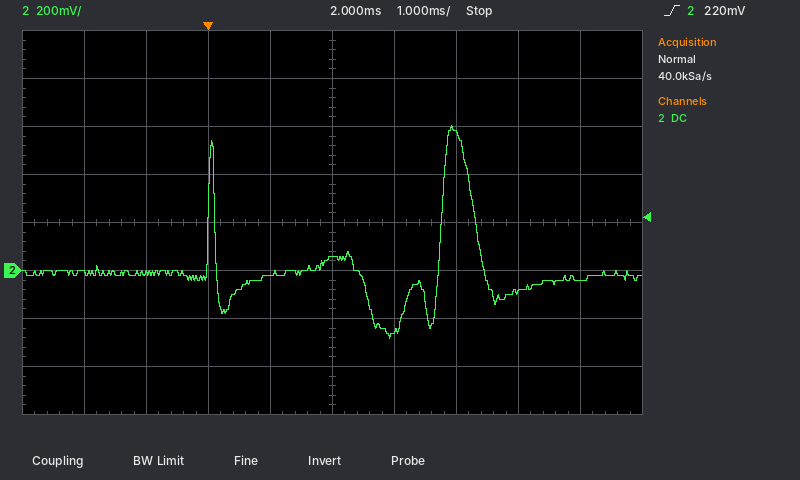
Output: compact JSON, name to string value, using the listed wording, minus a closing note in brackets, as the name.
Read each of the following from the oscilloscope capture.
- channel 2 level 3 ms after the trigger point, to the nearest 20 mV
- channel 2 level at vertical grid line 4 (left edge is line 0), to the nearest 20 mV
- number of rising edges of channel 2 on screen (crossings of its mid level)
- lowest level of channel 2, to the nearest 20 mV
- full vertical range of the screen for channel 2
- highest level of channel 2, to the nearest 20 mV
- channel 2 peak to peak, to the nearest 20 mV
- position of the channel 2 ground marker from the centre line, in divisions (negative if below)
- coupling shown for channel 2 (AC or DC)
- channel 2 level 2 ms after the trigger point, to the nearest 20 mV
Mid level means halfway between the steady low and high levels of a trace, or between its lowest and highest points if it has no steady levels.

{"channel 2 level 3 ms after the trigger point, to the nearest 20 mV": "-260 mV", "channel 2 level at vertical grid line 4 (left edge is line 0), to the nearest 20 mV": "-20 mV", "number of rising edges of channel 2 on screen": "2", "lowest level of channel 2, to the nearest 20 mV": "-280 mV", "full vertical range of the screen for channel 2": "1.6 V", "highest level of channel 2, to the nearest 20 mV": "600 mV", "channel 2 peak to peak, to the nearest 20 mV": "880 mV", "position of the channel 2 ground marker from the centre line, in divisions": "-1.0 div", "coupling shown for channel 2": "DC", "channel 2 level 2 ms after the trigger point, to the nearest 20 mV": "60 mV"}
